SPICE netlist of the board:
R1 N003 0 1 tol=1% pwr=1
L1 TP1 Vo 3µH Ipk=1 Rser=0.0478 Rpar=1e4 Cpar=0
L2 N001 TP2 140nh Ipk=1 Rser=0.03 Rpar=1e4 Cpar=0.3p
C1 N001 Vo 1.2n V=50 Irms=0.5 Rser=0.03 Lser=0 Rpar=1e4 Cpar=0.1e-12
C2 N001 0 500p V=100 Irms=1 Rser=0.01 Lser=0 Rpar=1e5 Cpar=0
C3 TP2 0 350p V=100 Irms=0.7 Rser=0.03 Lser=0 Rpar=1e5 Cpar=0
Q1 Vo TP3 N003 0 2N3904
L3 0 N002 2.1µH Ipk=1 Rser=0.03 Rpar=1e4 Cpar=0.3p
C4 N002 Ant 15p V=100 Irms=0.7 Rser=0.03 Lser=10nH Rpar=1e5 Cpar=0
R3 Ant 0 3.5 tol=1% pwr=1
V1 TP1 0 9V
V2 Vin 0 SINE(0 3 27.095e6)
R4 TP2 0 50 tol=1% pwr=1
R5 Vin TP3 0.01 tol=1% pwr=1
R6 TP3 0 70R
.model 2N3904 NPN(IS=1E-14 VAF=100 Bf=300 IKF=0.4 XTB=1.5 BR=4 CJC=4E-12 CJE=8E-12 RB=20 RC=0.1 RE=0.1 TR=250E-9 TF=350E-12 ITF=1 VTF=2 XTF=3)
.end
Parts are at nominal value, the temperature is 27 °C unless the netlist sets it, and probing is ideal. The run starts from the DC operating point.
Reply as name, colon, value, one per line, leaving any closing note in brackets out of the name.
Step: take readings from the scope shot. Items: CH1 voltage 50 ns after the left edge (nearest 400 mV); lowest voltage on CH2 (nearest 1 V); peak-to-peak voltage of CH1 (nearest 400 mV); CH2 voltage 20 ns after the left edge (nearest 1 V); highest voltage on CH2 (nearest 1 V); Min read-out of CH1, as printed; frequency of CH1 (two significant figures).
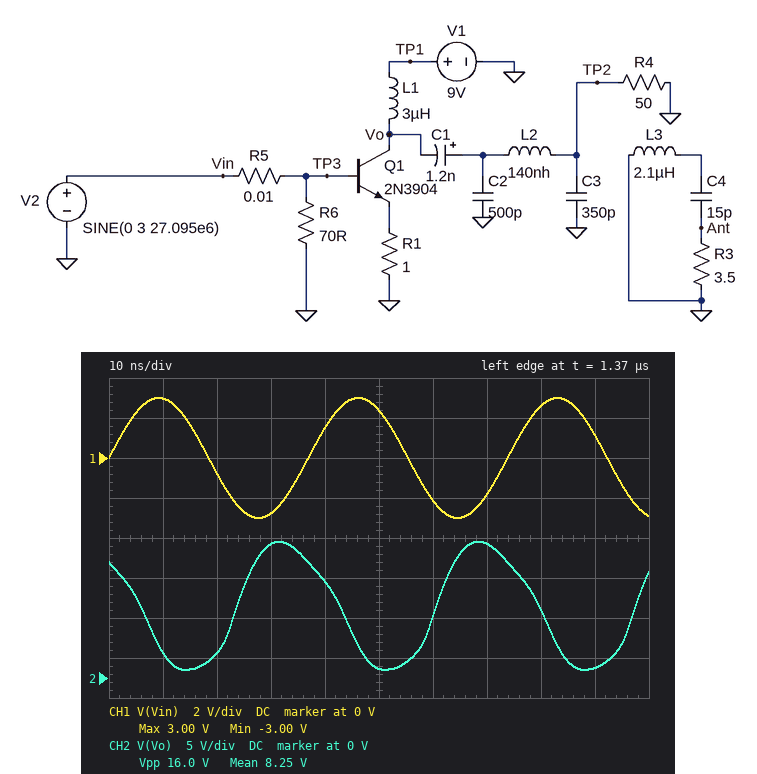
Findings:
CH1 voltage 50 ns after the left edge: 2.4 V
lowest voltage on CH2: 1 V
peak-to-peak voltage of CH1: 6.0 V
CH2 voltage 20 ns after the left edge: 3 V
highest voltage on CH2: 17 V
Min read-out of CH1, as printed: -3.00 V
frequency of CH1: 27 MHz
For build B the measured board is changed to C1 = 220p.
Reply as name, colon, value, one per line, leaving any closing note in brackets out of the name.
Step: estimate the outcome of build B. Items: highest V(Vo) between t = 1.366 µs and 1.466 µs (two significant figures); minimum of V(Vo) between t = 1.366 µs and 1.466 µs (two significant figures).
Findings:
highest V(Vo) between t = 1.366 µs and 1.466 µs: 19 V
minimum of V(Vo) between t = 1.366 µs and 1.466 µs: 520 mV
